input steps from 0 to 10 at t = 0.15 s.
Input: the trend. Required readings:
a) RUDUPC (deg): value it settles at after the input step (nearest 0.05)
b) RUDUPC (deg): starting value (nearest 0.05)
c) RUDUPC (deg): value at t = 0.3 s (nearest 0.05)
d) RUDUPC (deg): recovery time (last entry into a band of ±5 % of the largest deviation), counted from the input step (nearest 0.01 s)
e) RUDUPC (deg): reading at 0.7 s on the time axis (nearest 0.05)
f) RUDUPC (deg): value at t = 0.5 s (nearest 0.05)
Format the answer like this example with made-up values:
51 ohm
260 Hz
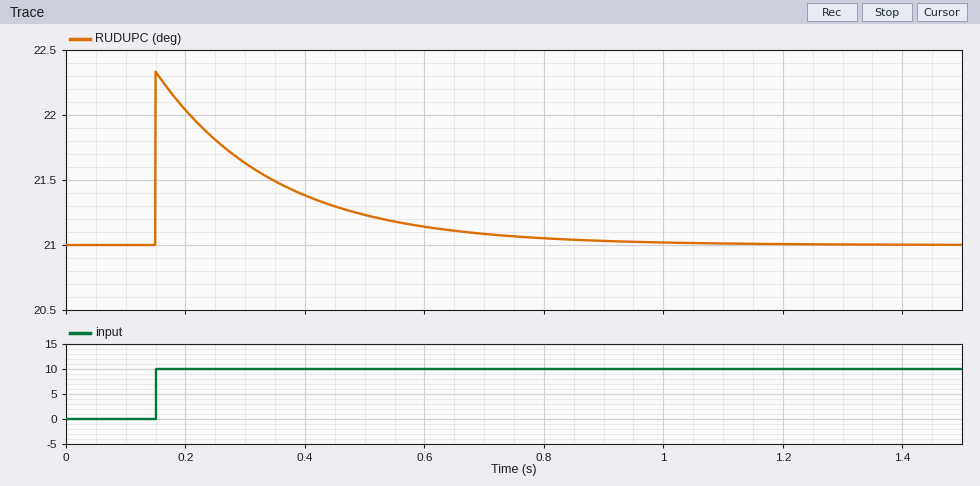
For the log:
21.00
21.00
21.65
0.60 s
21.10
21.25
